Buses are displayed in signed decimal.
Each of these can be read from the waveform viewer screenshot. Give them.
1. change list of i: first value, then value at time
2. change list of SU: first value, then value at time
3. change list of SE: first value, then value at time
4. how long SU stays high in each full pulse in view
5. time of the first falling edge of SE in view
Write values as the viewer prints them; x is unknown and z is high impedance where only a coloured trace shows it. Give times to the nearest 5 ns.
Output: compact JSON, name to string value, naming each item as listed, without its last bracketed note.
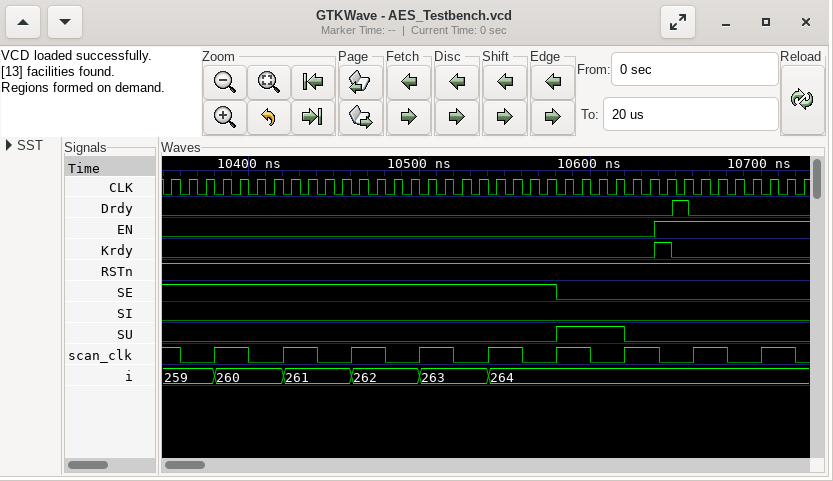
{"change list of i: first value, then value at time": "259, 260 at 10380 ns, 261 at 10420 ns, 262 at 10460 ns, 263 at 10500 ns, 264 at 10540 ns", "change list of SU: first value, then value at time": "0, 1 at 10580 ns, 0 at 10620 ns", "change list of SE: first value, then value at time": "1, 0 at 10580 ns", "how long SU stays high in each full pulse in view": "40 ns", "time of the first falling edge of SE in view": "10580 ns"}
